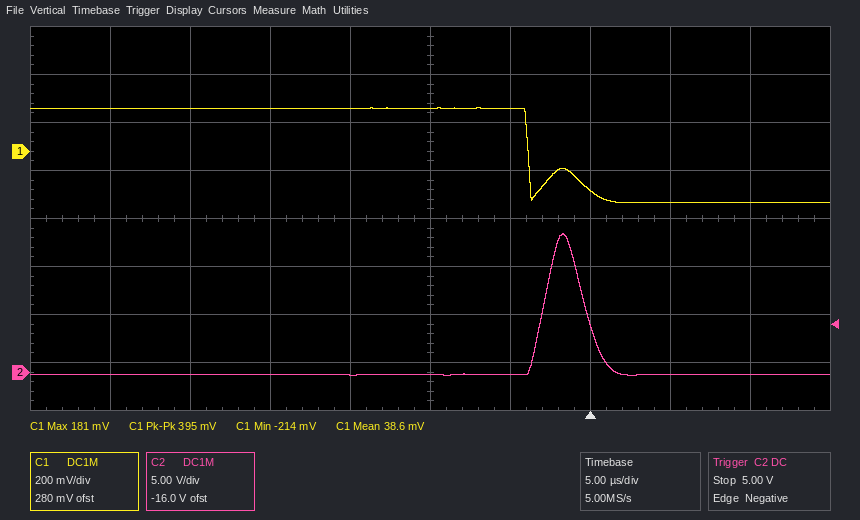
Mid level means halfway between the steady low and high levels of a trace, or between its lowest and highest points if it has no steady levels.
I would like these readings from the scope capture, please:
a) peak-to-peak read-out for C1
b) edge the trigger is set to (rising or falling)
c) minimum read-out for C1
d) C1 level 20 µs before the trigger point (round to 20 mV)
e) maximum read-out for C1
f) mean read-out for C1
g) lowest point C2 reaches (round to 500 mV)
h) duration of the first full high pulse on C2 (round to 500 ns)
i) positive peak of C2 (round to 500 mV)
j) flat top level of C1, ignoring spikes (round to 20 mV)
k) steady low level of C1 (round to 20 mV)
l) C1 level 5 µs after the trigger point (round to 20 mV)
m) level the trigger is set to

395 mV
falling
-214 mV
180 mV
181 mV
38.6 mV
-500 mV
2.5 µs
14.5 V
180 mV
-220 mV
-220 mV
5.00 V
